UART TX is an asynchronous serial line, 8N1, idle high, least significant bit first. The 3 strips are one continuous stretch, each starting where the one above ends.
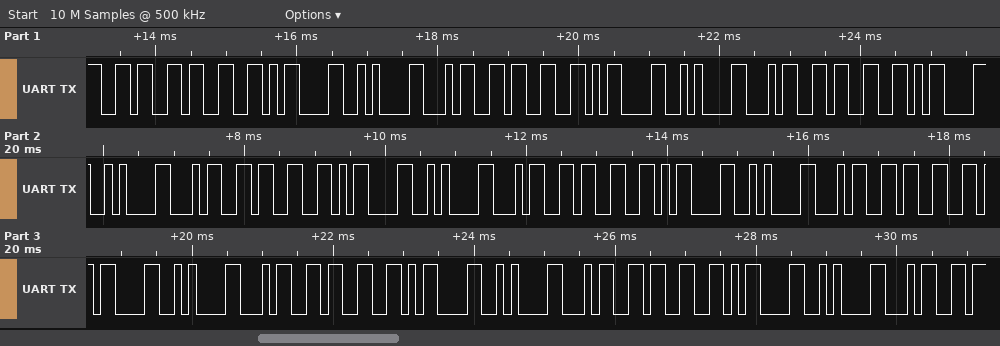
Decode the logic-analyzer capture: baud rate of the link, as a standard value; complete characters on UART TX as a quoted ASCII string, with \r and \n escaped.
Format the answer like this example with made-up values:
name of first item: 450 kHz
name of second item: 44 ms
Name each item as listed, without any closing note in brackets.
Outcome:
baud rate of the link, as a standard value: 9600 baud
complete characters on UART TX as a quoted ASCII string, with \r and \n escaped: "63\r\n43\r\n43\r\n43\r\n43\r\n43\r\n43\r\n43\r\n4"
